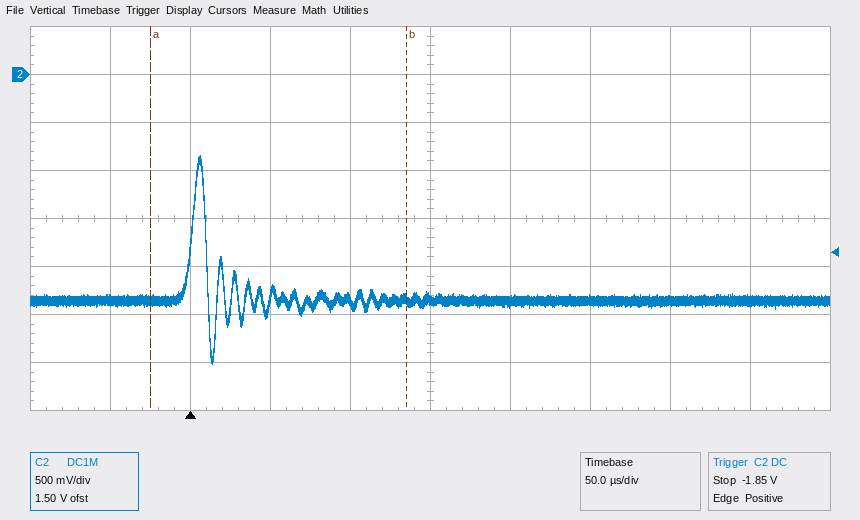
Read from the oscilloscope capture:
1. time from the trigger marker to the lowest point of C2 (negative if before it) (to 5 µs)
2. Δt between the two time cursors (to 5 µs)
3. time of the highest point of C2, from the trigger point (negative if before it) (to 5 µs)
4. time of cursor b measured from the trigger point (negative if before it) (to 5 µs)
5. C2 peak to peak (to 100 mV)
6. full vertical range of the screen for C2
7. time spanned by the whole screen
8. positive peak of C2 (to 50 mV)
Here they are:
+15 µs
160 µs
+5 µs
+135 µs
2.20 V
4 V
500 µs
-850 mV
